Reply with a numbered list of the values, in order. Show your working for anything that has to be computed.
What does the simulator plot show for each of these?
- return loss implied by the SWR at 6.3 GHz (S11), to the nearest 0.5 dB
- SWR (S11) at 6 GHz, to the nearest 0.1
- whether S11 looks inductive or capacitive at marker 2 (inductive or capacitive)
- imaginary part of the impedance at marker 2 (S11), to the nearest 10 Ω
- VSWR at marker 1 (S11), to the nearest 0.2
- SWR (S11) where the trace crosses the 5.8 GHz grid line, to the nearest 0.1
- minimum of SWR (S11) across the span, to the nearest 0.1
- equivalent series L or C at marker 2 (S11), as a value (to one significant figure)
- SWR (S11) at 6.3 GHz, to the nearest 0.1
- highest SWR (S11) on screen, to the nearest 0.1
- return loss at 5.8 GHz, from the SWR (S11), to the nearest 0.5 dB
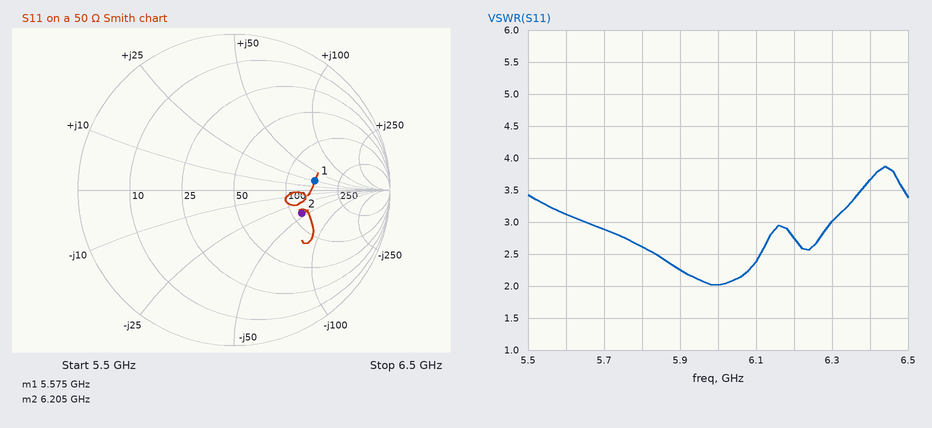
1. −20 log10((3 − 1)/(3 + 1)) ≈ 6.0 dB
2. 2.0
3. capacitive
4. -40 Ω
5. 3.2
6. 2.6
7. 2.0
8. C = 1/(2π × 6.205 GHz × 40 Ω) ≈ 641 fF, so 600 fF to one significant figure
9. 3.0
10. 3.9
11. −20 log10((2.6 − 1)/(2.6 + 1)) ≈ 7.0 dB
